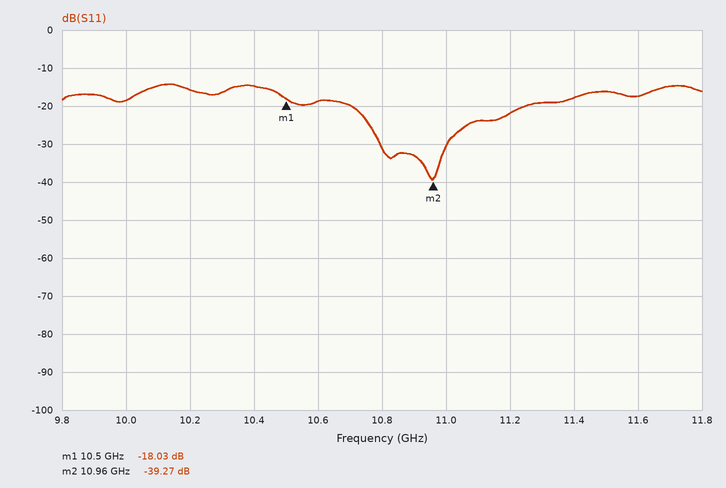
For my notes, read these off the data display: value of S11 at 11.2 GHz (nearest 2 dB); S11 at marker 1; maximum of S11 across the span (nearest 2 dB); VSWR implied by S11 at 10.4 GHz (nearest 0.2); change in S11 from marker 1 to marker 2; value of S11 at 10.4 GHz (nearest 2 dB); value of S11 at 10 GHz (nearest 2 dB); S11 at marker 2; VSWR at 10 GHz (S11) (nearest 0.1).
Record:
-22 dB
-18.03 dB
-14 dB
1.4
-21.24 dB
-14 dB
-18 dB
-39.27 dB
1.3
